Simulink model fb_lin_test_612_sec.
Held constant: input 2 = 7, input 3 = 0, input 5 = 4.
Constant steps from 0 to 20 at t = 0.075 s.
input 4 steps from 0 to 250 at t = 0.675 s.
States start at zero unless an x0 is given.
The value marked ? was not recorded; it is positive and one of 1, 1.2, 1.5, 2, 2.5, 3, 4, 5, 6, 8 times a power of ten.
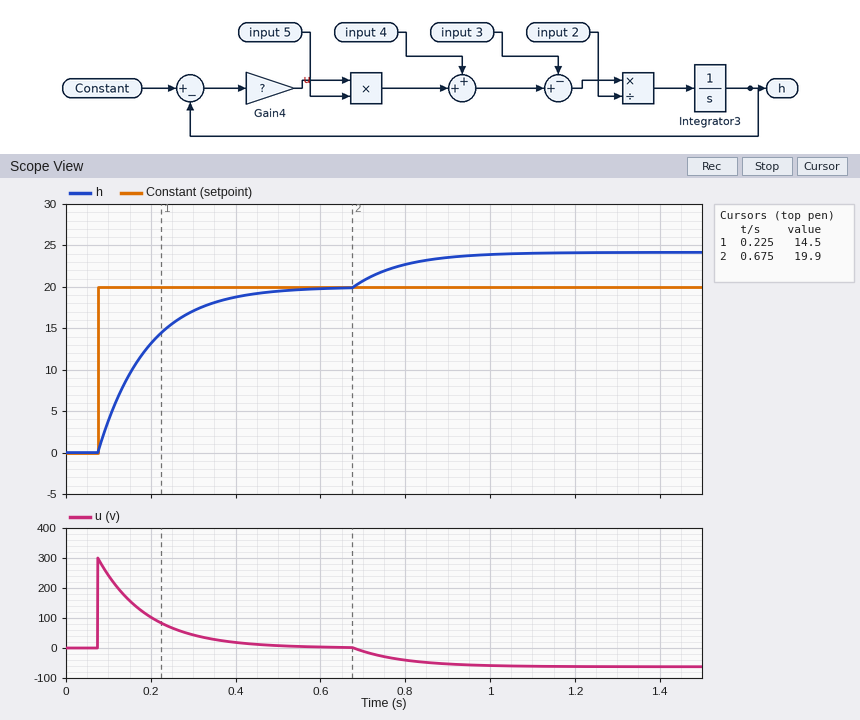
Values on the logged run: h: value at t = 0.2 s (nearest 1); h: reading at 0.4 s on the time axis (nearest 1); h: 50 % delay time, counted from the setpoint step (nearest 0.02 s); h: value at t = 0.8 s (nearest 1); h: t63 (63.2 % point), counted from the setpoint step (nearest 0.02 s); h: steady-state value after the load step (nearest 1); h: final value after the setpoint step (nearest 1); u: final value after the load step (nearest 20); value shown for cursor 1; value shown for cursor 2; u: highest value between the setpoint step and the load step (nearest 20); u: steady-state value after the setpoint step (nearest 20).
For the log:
13
19
0.08 s
23
0.12 s
24
20
-60
14.5
19.9
300
0
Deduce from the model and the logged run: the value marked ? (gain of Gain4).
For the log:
15
